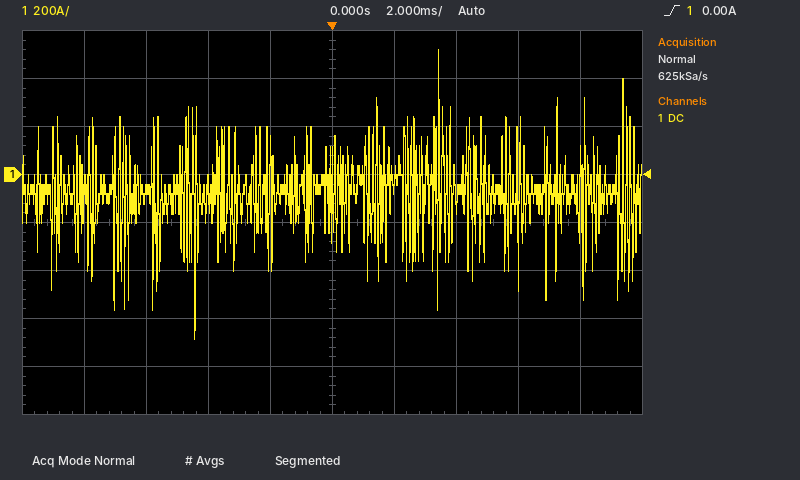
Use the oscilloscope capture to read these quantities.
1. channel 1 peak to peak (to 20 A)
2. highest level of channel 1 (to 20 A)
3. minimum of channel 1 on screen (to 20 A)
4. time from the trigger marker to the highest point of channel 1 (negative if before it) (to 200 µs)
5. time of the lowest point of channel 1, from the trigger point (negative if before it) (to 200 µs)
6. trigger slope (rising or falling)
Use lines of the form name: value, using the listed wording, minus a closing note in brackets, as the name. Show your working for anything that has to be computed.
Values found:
channel 1 peak to peak: 520 A − (-680 A) = 1.20 kA
highest level of channel 1: 520 A
minimum of channel 1 on screen: -680 A
time from the trigger marker to the highest point of channel 1 (negative if before it): +3.4 ms
time of the lowest point of channel 1, from the trigger point (negative if before it): -4.4 ms
trigger slope: rising
